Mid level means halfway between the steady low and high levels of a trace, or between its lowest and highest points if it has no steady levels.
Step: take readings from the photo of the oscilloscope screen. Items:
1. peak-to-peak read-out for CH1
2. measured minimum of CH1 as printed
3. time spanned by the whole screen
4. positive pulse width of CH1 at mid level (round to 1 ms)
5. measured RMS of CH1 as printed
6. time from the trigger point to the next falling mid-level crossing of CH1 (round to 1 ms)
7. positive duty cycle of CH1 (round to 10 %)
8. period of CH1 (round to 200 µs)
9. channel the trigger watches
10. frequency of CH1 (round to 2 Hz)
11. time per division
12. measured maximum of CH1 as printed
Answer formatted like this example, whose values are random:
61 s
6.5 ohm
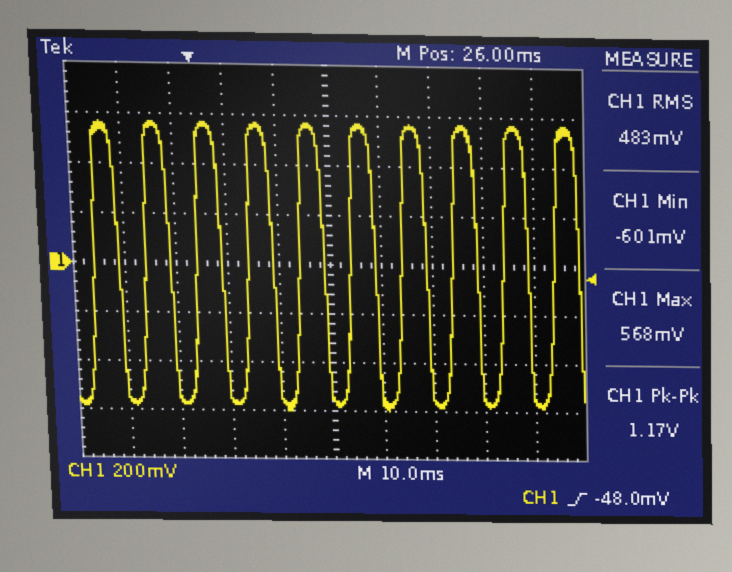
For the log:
1.17 V
-601 mV
100 ms
5 ms
483 mV
5 ms
50 %
10.0 ms
CH1
100 Hz
10 ms
568 mV
